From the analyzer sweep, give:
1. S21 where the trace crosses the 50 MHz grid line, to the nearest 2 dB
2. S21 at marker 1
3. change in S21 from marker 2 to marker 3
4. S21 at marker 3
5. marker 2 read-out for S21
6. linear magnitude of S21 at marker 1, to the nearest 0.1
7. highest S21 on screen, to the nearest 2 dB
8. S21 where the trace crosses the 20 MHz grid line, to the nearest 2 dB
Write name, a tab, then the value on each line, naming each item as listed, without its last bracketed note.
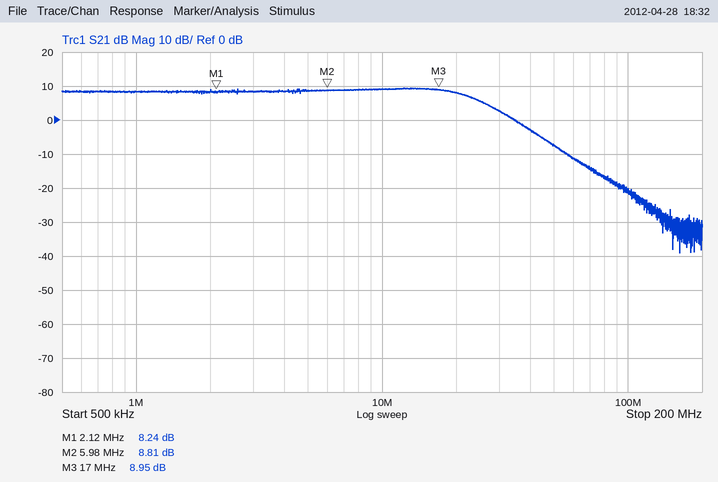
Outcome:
S21 where the trace crosses the 50 MHz grid line, to the nearest 2 dB	-8 dB
S21 at marker 1	8.24 dB
change in S21 from marker 2 to marker 3	0.14 dB
S21 at marker 3	8.95 dB
marker 2 read-out for S21	8.81 dB
linear magnitude of S21 at marker 1, to the nearest 0.1	2.6
highest S21 on screen, to the nearest 2 dB	10 dB
S21 where the trace crosses the 20 MHz grid line, to the nearest 2 dB	8 dB
